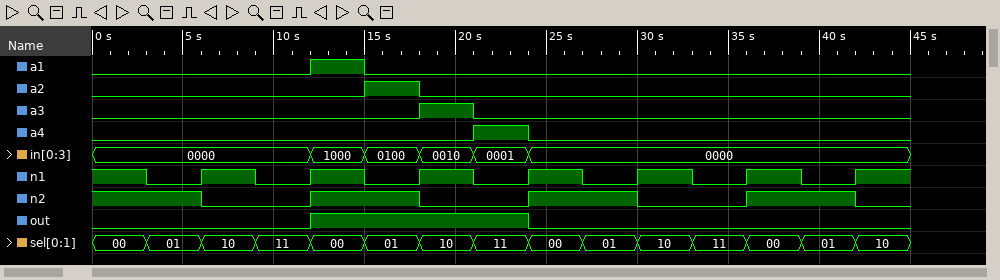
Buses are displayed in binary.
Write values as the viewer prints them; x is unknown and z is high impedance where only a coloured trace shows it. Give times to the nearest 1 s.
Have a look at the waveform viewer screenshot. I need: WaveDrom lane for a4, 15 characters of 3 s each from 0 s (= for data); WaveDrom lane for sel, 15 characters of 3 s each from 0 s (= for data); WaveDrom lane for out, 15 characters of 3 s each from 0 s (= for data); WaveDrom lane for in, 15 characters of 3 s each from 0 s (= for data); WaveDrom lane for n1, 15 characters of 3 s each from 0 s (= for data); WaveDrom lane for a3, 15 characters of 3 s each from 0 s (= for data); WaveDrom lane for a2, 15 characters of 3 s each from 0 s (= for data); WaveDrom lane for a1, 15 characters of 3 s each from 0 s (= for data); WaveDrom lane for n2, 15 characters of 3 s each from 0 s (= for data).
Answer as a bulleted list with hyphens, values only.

- {name: 'a4', wave: '0......10......'}
- {name: 'sel', wave: '===============', data: '00 01 10 11 00 01 10 11 00 01 10 11 00 01 10'}
- {name: 'out', wave: '0...1...0......'}
- {name: 'in', wave: '=...=====......', data: '0000 1000 0100 0010 0001 0000'}
- {name: 'n1', wave: '101010101010101'}
- {name: 'a3', wave: '0.....10.......'}
- {name: 'a2', wave: '0....10........'}
- {name: 'a1', wave: '0...10.........'}
- {name: 'n2', wave: '1.0.1.0.1.0.1.0'}
